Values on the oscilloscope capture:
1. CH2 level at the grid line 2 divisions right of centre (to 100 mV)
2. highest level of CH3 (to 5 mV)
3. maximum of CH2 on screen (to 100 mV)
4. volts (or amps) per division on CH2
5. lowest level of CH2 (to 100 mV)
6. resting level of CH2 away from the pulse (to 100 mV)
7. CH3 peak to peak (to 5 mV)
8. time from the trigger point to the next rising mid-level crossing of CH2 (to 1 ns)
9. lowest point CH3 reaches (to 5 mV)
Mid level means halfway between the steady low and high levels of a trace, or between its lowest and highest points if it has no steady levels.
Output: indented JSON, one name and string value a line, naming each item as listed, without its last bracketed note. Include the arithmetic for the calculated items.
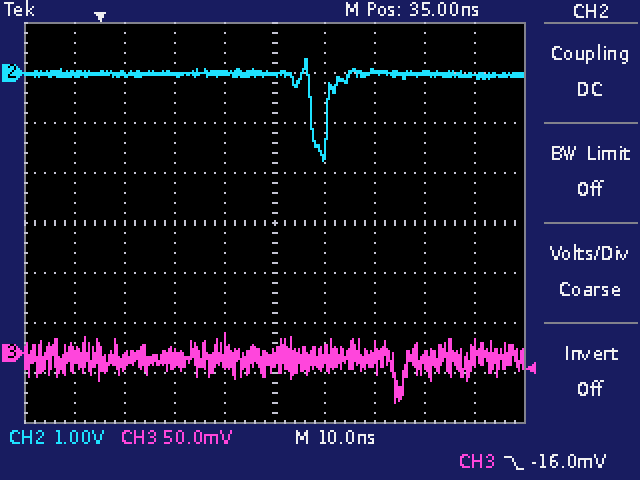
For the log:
{
  "CH2 level at the grid line 2 divisions right of centre": "0.0 V",
  "highest level of CH3": "20 mV",
  "maximum of CH2 on screen": "300 mV",
  "volts (or amps) per division on CH2": "1 V",
  "lowest level of CH2": "-1.8 V",
  "resting level of CH2 away from the pulse": "0.0 V",
  "CH3 peak to peak": "20 mV − (-50 mV) = 70 mV",
  "time from the trigger point to the next rising mid-level crossing of CH2": "46 ns",
  "lowest point CH3 reaches": "-50 mV"
}
